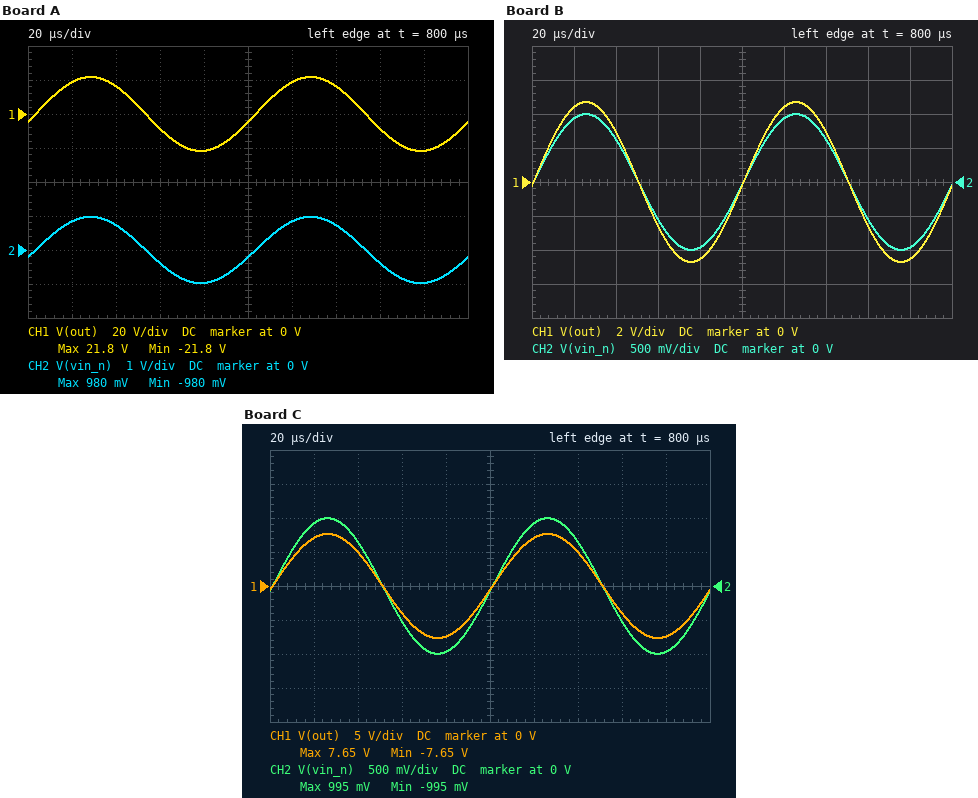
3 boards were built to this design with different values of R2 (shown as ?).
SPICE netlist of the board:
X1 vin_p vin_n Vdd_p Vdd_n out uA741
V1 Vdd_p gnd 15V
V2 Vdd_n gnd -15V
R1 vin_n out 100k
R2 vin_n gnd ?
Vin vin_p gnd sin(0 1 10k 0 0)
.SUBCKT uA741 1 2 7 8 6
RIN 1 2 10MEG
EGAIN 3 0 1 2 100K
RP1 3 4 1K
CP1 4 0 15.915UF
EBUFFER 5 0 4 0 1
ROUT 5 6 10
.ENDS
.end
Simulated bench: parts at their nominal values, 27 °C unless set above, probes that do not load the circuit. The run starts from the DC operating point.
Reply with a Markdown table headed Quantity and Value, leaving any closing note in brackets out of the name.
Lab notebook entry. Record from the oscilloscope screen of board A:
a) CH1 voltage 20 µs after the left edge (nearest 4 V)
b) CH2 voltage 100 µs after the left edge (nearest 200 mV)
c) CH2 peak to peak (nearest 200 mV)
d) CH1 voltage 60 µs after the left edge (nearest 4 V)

| Quantity | Value |
|---|---|
| CH1 voltage 20 µs after the left edge | 20 V |
| CH2 voltage 100 µs after the left edge | -200 mV |
| CH2 peak to peak | 2.0 V |
| CH1 voltage 60 µs after the left edge | -8 V |
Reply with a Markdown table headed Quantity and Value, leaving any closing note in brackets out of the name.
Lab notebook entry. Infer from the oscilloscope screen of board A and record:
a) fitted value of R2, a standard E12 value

| Quantity | Value |
|---|---|
| fitted value of R2, a standard E12 value | 4.7 kΩ |
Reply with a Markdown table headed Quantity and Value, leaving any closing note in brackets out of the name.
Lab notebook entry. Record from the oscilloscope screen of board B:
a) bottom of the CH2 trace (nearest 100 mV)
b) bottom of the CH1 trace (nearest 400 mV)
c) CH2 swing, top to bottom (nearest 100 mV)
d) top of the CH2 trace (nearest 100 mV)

| Quantity | Value |
|---|---|
| bottom of the CH2 trace | -1.0 V |
| bottom of the CH1 trace | -4.8 V |
| CH2 swing, top to bottom | 2.0 V |
| top of the CH2 trace | 1.0 V |
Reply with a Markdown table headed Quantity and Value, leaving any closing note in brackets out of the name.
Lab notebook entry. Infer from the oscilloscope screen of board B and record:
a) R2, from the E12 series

| Quantity | Value |
|---|---|
| R2, from the E12 series | 27 kΩ |
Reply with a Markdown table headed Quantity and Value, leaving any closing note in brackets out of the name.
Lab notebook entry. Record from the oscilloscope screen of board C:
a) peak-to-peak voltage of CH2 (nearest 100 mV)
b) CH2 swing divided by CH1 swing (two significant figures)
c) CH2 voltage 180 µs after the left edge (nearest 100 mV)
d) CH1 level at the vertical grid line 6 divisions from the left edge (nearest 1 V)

| Quantity | Value |
|---|---|
| peak-to-peak voltage of CH2 | 2.0 V |
| CH2 swing divided by CH1 swing | 0.13 |
| CH2 voltage 180 µs after the left edge | -1.0 V |
| CH1 level at the vertical grid line 6 divisions from the left edge | 7 V |
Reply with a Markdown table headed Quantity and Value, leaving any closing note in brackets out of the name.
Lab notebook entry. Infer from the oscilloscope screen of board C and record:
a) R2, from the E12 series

| Quantity | Value |
|---|---|
| R2, from the E12 series | 15 kΩ |
